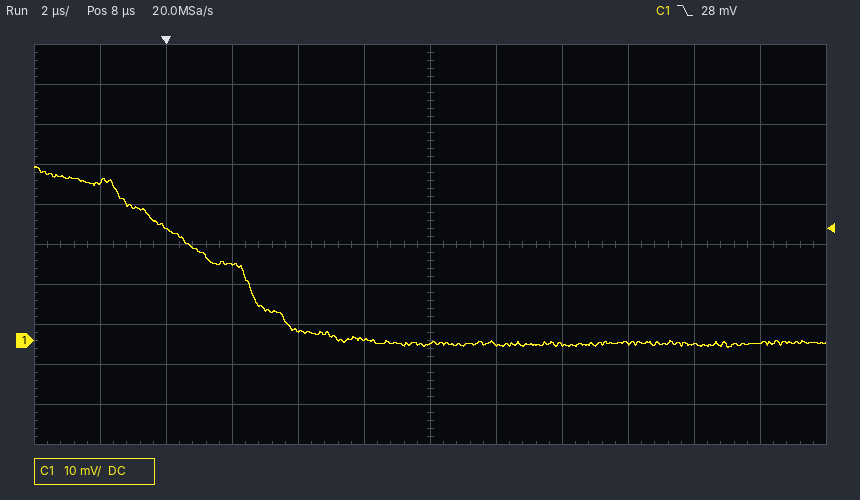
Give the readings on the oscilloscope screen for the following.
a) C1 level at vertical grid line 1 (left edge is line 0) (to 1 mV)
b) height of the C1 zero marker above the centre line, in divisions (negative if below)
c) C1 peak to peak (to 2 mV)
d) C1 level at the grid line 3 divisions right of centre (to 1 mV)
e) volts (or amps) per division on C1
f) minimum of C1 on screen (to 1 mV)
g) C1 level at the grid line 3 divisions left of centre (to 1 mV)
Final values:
40 mV
-2.4 div
46 mV
-1 mV
10 mV
-2 mV
19 mV
